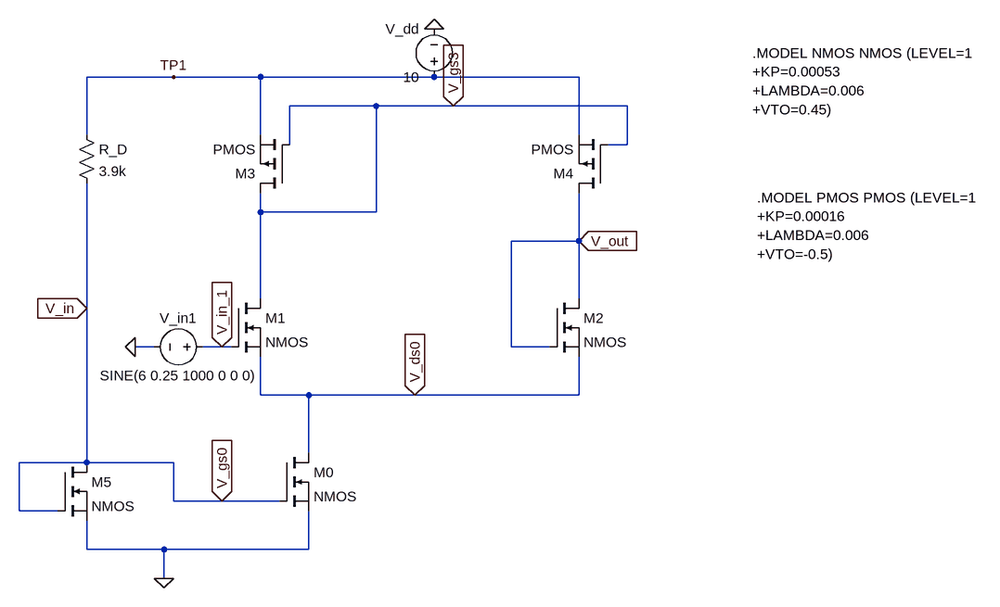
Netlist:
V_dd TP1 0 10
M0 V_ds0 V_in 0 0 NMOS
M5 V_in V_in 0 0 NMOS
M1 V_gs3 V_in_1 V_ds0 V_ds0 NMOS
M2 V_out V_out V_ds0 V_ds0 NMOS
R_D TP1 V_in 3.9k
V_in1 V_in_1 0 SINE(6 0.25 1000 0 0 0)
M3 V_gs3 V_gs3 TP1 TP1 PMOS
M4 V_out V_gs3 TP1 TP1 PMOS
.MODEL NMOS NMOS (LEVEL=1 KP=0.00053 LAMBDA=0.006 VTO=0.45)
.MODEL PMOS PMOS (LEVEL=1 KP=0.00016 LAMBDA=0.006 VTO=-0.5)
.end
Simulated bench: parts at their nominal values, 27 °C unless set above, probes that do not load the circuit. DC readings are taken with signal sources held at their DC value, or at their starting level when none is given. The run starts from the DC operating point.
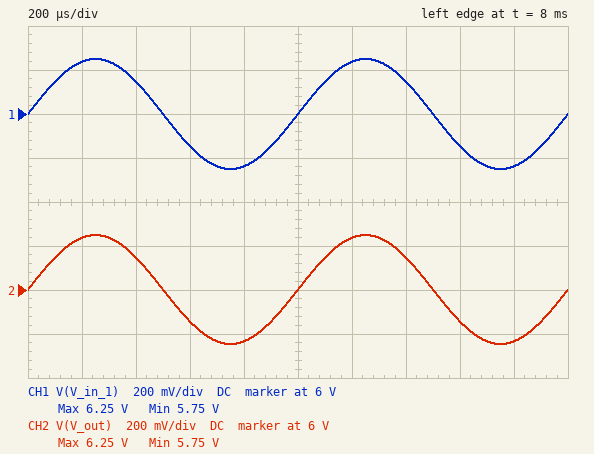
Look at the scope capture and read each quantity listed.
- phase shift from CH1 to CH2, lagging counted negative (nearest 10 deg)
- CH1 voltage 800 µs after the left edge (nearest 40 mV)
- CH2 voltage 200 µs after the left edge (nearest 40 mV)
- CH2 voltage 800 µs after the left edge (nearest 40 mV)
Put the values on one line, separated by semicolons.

0 deg; 5.76 V; 6.24 V; 5.76 V
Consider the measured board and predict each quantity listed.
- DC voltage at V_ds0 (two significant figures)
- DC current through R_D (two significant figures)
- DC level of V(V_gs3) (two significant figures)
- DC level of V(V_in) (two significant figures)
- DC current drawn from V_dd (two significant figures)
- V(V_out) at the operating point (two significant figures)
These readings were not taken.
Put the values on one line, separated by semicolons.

3.7 V; 1.8 mA; 6.2 V; 3.0 V; 3.6 mA; 6.0 V
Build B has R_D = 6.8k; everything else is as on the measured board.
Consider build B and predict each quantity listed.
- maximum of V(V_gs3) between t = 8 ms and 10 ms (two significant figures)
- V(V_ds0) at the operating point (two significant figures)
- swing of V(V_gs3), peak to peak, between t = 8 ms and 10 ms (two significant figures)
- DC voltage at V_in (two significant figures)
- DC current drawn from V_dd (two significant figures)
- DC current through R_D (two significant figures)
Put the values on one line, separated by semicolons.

6.9 V; 4.1 V; 5.7 mV; 2.5 V; 2.2 mA; 1.1 mA
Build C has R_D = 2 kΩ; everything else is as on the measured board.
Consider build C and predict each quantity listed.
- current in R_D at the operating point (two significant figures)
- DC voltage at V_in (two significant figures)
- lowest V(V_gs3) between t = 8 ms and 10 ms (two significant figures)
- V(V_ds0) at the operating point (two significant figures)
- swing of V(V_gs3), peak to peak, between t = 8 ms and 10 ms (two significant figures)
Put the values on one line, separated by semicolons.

3.1 mA; 3.8 V; 5.2 V; 3.1 V; 58 mV
